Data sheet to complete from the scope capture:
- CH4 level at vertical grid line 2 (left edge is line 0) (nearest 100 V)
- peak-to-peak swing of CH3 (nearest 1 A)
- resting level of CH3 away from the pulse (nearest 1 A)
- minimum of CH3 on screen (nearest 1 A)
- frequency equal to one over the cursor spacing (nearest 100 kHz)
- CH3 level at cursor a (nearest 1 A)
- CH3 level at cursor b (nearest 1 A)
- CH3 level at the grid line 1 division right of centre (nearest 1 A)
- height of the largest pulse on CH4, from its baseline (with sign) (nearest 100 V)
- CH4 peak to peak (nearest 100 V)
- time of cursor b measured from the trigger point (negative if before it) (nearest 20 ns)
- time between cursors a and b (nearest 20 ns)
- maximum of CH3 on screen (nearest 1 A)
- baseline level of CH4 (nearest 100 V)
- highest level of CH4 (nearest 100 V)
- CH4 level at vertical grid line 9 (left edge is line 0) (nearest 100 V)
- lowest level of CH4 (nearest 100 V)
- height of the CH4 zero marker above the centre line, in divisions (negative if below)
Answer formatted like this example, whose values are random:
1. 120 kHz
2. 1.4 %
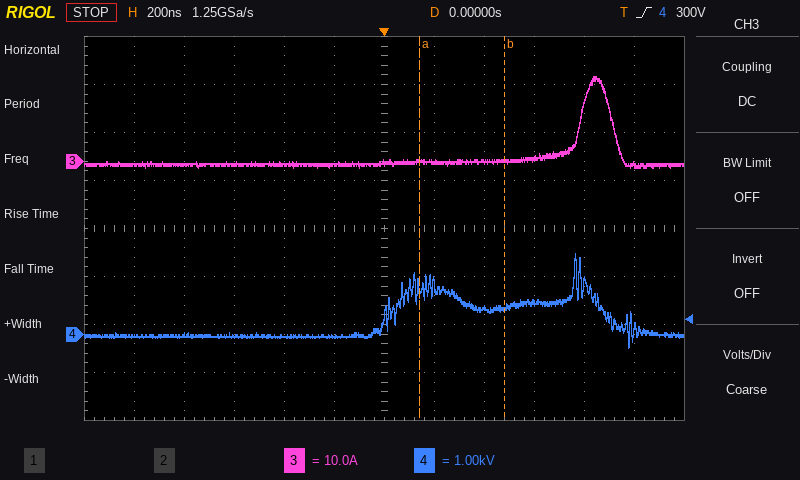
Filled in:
1. 0.0 kV
2. 19 A
3. -1 A
4. -1 A
5. 2.9 MHz
6. 0 A
7. 0 A
8. 0 A
9. +1.7 kV
10. 2.0 kV
11. +480 ns
12. 340 ns
13. 18 A
14. 0.0 kV
15. 1.7 kV
16. 700 V
17. -300 V
18. -2.2 div
